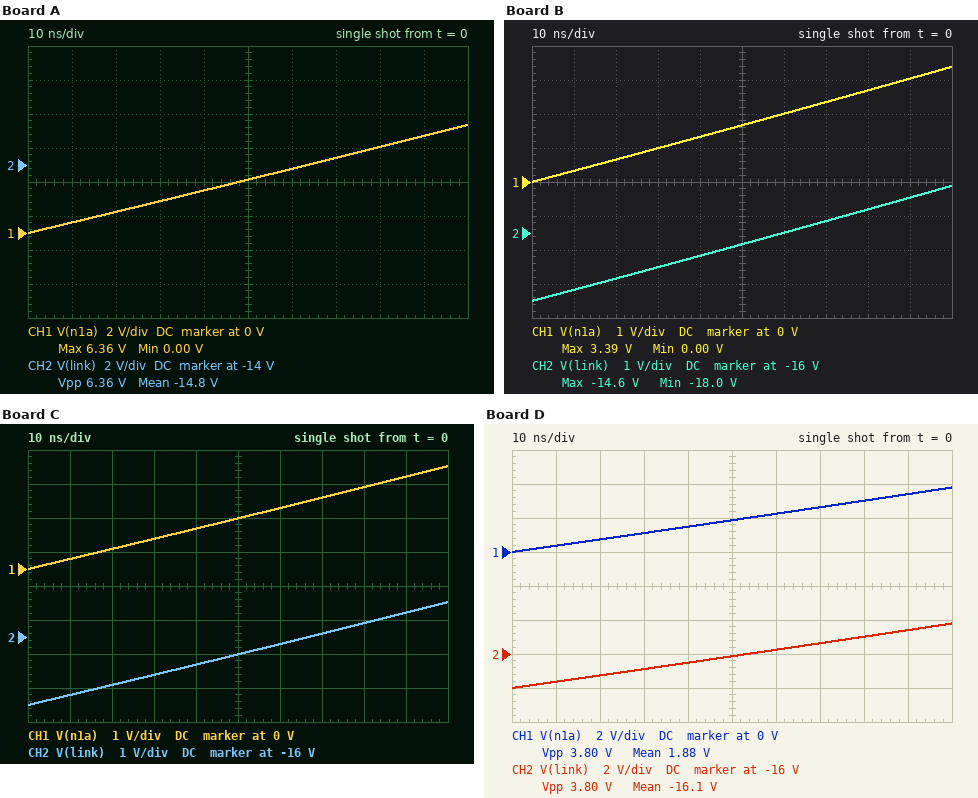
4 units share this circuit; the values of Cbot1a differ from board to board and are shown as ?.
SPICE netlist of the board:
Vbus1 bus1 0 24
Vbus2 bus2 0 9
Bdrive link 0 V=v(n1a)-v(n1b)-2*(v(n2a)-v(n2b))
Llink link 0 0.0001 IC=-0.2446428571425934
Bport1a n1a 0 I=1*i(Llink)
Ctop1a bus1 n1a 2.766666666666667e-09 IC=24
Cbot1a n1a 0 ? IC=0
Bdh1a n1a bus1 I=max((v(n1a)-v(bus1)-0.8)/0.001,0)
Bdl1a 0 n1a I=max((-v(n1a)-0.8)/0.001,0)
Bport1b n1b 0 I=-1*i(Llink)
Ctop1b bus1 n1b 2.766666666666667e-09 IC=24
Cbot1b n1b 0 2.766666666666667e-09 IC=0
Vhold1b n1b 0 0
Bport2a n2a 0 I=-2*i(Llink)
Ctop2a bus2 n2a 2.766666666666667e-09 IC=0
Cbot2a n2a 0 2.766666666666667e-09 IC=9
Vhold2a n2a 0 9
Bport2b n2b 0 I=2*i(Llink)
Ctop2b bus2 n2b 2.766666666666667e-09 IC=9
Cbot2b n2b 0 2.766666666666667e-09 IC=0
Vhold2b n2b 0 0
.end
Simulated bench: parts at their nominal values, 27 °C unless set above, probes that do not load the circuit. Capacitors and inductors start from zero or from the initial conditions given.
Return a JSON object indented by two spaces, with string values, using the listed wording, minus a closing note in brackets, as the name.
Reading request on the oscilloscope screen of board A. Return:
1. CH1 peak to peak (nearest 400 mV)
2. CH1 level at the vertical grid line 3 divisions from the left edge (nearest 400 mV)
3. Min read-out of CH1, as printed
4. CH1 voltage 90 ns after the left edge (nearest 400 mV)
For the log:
{
  "CH1 peak to peak": "6.4 V",
  "CH1 level at the vertical grid line 3 divisions from the left edge": "2.0 V",
  "Min read-out of CH1, as printed": "0.00 V",
  "CH1 voltage 90 ns after the left edge": "5.6 V"
}
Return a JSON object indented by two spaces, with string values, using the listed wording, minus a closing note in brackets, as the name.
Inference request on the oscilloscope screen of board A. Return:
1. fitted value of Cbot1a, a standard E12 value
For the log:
{
  "fitted value of Cbot1a, a standard E12 value": "1.2 nF"
}
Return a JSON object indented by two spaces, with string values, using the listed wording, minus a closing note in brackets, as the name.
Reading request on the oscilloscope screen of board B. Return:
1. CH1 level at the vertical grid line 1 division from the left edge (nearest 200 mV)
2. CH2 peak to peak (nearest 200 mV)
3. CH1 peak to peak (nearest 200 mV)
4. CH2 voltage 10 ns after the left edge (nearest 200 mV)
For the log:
{
  "CH1 level at the vertical grid line 1 division from the left edge": "400 mV",
  "CH2 peak to peak": "3.4 V",
  "CH1 peak to peak": "3.4 V",
  "CH2 voltage 10 ns after the left edge": "-17.6 V"
}
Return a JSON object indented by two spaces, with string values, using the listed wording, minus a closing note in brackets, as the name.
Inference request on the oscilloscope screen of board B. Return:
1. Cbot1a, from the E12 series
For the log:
{
  "Cbot1a, from the E12 series": "4.7 nF"
}
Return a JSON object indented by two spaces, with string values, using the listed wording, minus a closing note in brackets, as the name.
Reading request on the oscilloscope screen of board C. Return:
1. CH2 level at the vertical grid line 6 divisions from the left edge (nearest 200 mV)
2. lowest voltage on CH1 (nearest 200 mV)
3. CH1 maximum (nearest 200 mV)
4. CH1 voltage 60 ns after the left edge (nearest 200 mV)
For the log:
{
  "CH2 level at the vertical grid line 6 divisions from the left edge": "-16.2 V",
  "lowest voltage on CH1": "0 V",
  "CH1 maximum": "3.0 V",
  "CH1 voltage 60 ns after the left edge": "1.8 V"
}
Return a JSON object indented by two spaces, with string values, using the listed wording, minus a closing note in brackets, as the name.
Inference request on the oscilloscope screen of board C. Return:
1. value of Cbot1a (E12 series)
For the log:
{
  "value of Cbot1a": "5.6 nF"
}
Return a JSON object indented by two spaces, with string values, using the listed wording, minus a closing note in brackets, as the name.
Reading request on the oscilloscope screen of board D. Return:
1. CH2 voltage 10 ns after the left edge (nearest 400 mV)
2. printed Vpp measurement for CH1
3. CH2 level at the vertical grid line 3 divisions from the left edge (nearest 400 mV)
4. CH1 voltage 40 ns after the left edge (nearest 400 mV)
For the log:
{
  "CH2 voltage 10 ns after the left edge": "-17.6 V",
  "printed Vpp measurement for CH1": "3.80 V",
  "CH2 level at the vertical grid line 3 divisions from the left edge": "-16.8 V",
  "CH1 voltage 40 ns after the left edge": "1.6 V"
}
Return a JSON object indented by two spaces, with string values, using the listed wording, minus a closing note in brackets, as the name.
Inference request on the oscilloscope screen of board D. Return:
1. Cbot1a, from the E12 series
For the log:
{
  "Cbot1a, from the E12 series": "3.9 nF"
}
